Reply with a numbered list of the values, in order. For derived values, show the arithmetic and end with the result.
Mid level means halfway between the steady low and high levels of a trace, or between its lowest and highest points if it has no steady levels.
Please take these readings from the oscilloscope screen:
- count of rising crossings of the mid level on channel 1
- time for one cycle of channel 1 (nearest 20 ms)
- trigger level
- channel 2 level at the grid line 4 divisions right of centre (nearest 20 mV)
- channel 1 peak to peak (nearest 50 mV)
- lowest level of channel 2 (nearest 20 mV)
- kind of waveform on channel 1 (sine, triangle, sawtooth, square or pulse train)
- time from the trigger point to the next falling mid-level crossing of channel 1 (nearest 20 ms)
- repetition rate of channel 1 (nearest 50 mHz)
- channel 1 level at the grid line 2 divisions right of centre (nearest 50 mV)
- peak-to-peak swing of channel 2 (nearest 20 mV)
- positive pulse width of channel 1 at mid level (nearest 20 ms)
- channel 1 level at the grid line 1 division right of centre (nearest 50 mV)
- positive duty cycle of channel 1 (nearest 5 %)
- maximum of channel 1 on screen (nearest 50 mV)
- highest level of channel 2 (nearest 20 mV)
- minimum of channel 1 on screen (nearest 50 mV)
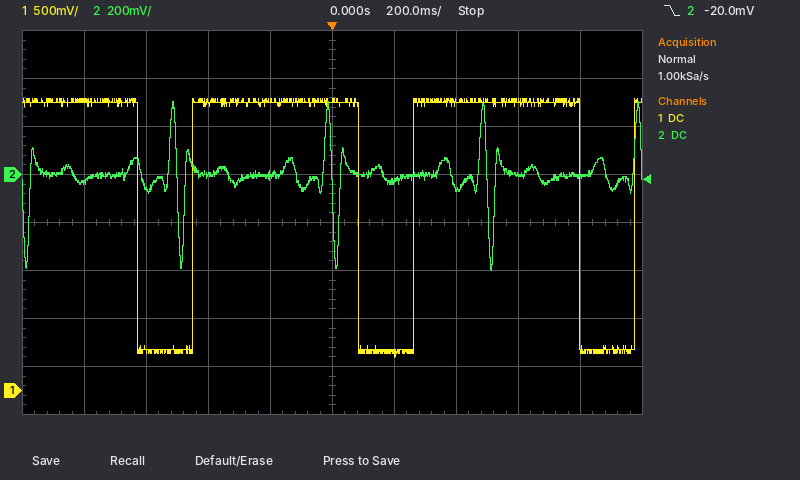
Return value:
1. 3
2. 720 ms
3. -20.0 mV
4. 0 mV
5. 3.05 V − (350 mV) = 2.70 V
6. -400 mV
7. pulse train
8. 80 ms
9. 1 / 720 ms ≈ 1.39 Hz, so 1.40 Hz to the nearest 50 mHz
10. 3.00 V
11. 300 mV − (-400 mV) = 700 mV
12. 540 ms
13. 400 mV
14. 540 ms / 720 ms ≈ 75 %
15. 3.05 V
16. 300 mV
17. 350 mV
